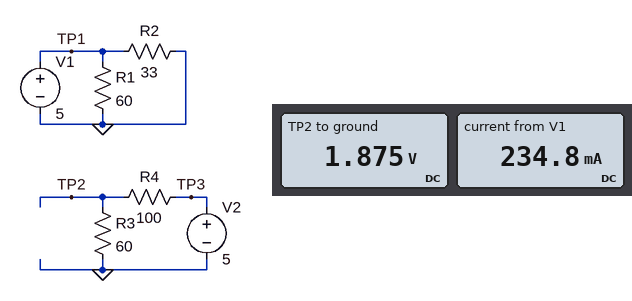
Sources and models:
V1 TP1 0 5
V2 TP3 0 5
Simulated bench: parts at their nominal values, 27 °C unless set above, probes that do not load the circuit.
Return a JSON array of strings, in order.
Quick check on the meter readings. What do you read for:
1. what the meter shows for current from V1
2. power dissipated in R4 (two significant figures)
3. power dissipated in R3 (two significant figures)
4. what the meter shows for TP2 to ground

["234.8 mA", "98 mW", "59 mW", "1.875 V"]
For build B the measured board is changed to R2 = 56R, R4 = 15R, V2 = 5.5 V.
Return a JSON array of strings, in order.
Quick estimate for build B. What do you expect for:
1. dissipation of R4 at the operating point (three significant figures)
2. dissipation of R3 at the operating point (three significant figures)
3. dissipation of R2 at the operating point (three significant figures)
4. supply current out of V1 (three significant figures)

["80.7 mW", "323 mW", "446 mW", "173 mA"]
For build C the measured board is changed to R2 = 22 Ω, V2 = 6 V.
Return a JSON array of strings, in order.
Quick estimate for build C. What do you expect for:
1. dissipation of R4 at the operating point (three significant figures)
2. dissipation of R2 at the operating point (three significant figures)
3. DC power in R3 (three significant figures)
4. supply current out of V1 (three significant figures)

["141 mW", "1.14 W", "84.4 mW", "311 mA"]
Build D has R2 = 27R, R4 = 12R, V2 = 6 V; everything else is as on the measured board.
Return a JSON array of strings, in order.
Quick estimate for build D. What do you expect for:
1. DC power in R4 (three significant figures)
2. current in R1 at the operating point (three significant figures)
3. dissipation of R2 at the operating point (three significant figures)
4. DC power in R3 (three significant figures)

["83.3 mW", "83.3 mA", "926 mW", "417 mW"]
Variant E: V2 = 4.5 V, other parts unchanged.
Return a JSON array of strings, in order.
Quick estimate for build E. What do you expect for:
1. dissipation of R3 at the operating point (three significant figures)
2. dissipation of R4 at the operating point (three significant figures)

["47.5 mW", "79.1 mW"]
